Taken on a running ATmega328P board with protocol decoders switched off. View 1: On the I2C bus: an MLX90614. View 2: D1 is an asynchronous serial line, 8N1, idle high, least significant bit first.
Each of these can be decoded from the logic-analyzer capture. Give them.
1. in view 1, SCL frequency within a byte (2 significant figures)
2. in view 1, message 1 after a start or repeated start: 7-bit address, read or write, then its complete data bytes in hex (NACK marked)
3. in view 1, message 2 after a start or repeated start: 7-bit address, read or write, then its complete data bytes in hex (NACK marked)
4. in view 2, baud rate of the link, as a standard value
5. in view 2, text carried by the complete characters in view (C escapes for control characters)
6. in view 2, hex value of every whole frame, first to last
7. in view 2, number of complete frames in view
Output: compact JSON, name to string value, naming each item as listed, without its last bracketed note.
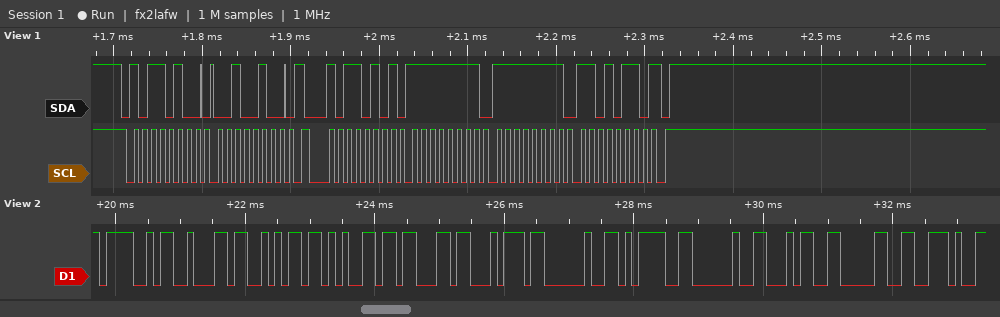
{"in view 1, SCL frequency within a byte": "100 kHz", "in view 1, message 1 after a start or repeated start: 7-bit address, read or write, then its complete data bytes in hex": "0x5A write: 24", "in view 1, message 2 after a start or repeated start: 7-bit address, read or write, then its complete data bytes in hex": "0x5A read: FF FF D6 NACK", "in view 2, baud rate of the link, as a standard value": "9600 baud", "in view 2, text carried by the complete characters in view": "\"Object = 40.\"", "in view 2, hex value of every whole frame, first to last": "4F 62 6A 65 63 74 20 3D 20 34 30 2E", "in view 2, number of complete frames in view": "12"}
